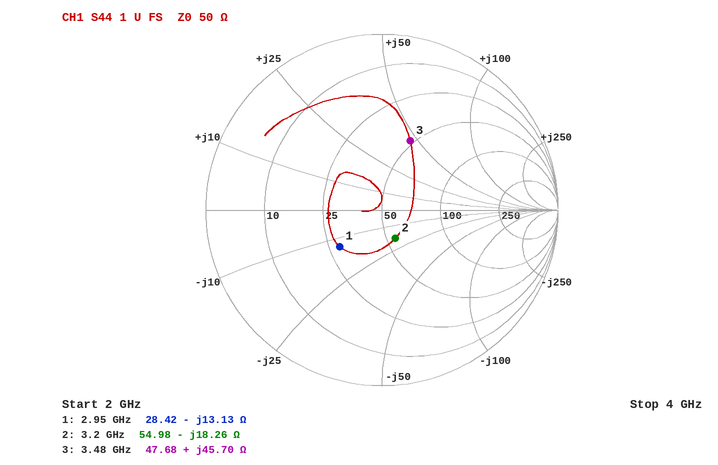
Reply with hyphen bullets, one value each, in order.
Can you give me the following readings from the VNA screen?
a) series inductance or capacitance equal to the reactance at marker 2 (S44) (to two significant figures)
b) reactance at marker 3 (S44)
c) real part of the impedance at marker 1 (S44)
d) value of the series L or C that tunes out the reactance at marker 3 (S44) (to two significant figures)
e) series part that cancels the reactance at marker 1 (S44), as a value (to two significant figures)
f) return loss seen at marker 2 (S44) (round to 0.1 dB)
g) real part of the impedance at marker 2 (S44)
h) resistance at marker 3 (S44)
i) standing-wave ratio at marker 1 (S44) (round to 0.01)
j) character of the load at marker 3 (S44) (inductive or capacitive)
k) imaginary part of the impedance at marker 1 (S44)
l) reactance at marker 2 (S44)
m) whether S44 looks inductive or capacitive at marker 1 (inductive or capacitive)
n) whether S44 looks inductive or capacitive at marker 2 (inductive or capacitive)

- 2.7 pF
- +45.70 Ω
- 28.42 Ω
- 1.0 pF
- 710 pH
- 15.0 dB
- 54.98 Ω
- 47.68 Ω
- 1.93
- inductive
- -13.13 Ω
- -18.26 Ω
- capacitive
- capacitive
